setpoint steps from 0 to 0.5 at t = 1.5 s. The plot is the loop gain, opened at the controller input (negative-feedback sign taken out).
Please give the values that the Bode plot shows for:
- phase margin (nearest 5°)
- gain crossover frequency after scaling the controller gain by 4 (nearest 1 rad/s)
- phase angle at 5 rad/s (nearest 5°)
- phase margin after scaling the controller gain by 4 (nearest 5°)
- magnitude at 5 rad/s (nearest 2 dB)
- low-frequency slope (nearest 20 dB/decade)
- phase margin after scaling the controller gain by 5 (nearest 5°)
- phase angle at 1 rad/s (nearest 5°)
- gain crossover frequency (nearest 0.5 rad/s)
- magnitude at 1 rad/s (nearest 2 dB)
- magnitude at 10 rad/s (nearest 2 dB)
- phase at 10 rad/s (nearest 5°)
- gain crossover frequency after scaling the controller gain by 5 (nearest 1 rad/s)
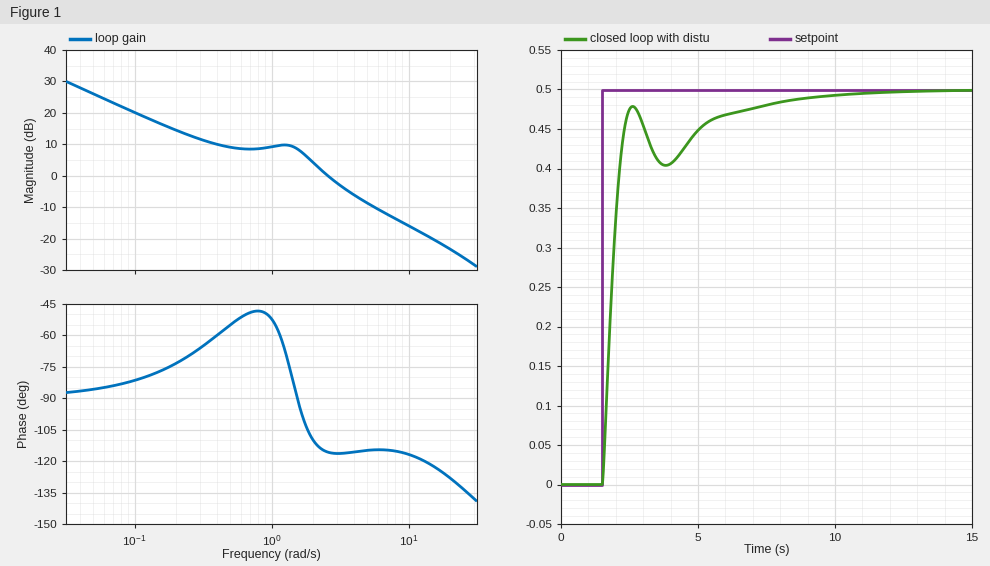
65°
7 rad/s
-115°
65°
-8 dB
-20 dB/decade
65°
-50°
2.5 rad/s
10 dB
-16 dB
-115°
8 rad/s
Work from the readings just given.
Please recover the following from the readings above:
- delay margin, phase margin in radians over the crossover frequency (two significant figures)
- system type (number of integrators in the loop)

0.45 s
1
